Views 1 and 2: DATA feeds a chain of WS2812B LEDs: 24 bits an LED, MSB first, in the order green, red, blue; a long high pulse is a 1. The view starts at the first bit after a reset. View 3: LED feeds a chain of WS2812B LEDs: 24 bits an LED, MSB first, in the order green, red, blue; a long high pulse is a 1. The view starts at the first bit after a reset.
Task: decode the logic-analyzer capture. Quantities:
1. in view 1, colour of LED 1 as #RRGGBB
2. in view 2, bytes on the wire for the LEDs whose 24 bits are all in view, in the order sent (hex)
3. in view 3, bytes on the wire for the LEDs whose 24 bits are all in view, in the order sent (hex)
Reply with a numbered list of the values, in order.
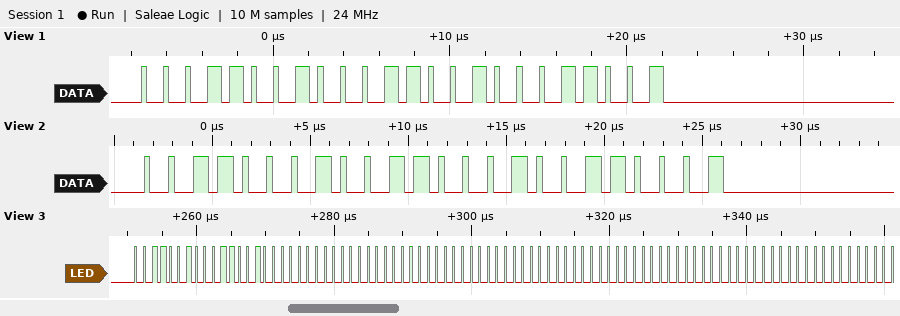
1. #191919
2. 31 31 31
3. 32 32 00 00 00 00 00 00 00
